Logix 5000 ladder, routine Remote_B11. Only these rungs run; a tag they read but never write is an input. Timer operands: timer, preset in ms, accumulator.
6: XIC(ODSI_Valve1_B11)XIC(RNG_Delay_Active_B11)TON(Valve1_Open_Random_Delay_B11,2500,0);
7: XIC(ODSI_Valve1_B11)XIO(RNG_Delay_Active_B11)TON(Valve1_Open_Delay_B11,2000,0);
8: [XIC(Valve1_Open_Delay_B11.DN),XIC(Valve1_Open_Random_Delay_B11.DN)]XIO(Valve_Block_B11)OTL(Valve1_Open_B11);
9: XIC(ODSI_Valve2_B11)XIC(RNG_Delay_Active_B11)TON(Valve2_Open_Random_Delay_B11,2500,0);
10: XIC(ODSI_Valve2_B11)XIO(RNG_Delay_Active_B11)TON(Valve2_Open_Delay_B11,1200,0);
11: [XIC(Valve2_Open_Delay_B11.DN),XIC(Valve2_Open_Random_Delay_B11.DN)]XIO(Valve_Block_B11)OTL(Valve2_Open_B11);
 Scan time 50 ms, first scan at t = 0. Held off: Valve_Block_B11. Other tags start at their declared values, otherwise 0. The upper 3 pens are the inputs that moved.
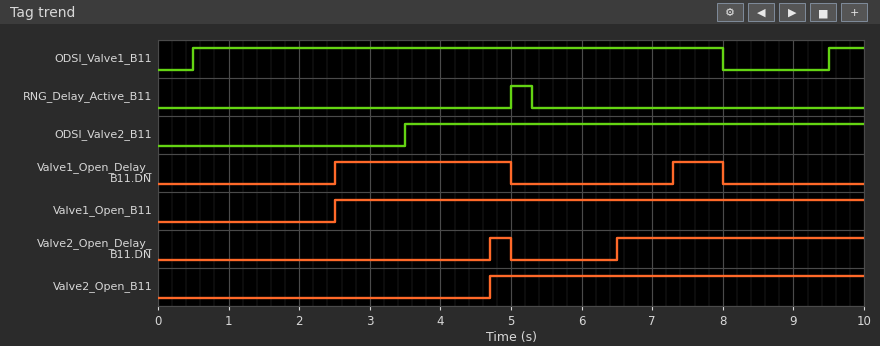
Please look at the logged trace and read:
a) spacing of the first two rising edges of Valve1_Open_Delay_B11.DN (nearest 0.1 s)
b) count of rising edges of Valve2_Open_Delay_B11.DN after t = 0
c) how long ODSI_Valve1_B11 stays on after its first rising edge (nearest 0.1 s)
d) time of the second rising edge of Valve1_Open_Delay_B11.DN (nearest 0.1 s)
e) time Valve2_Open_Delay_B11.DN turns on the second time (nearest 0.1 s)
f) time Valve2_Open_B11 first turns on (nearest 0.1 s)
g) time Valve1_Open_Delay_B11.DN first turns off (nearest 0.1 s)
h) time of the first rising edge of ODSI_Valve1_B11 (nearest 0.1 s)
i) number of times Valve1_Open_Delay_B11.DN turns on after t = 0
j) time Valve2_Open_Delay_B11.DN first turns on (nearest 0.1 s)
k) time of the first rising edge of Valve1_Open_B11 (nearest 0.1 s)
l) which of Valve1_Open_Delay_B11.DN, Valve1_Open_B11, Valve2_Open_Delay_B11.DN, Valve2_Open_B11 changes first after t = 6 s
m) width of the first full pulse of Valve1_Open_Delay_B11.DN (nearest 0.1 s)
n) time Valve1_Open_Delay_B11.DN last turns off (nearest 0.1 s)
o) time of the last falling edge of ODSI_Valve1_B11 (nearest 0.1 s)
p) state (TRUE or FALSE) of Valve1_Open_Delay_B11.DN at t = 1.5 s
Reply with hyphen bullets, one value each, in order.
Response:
- 4.8 s
- 2
- 7.5 s
- 7.3 s
- 6.5 s
- 4.7 s
- 5.0 s
- 0.5 s
- 2
- 4.7 s
- 2.5 s
- Valve2_Open_Delay_B11.DN
- 2.5 s
- 8.0 s
- 8.0 s
- FALSE
